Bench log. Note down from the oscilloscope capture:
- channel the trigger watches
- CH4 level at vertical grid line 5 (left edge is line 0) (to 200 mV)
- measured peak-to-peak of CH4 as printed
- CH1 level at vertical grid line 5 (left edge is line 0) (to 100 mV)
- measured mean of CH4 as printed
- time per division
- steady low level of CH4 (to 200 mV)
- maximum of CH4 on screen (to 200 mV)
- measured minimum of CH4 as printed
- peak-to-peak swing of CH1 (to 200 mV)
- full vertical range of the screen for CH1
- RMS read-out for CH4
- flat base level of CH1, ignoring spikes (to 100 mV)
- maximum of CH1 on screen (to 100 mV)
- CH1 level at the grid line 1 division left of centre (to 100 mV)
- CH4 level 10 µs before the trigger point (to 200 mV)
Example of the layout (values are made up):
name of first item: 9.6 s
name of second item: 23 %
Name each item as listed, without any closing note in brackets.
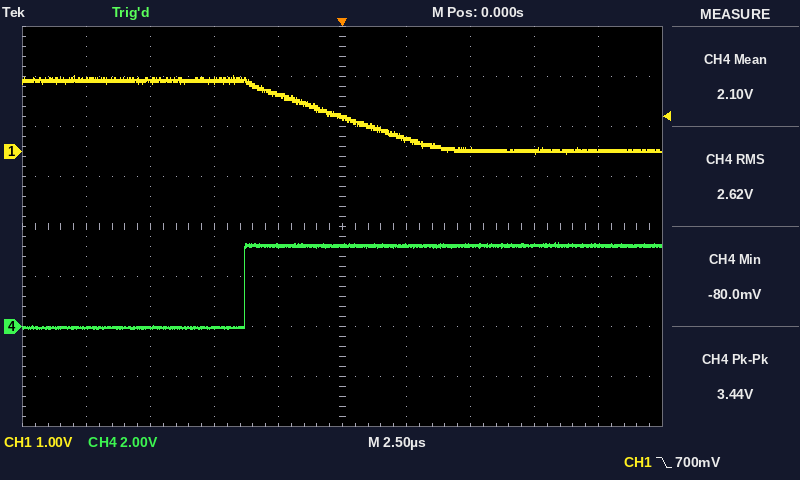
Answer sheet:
channel the trigger watches: CH1
CH4 level at vertical grid line 5 (left edge is line 0): 3.2 V
measured peak-to-peak of CH4 as printed: 3.44 V
CH1 level at vertical grid line 5 (left edge is line 0): 700 mV
measured mean of CH4 as printed: 2.10 V
time per division: 2.5 µs
steady low level of CH4: 0.0 V
maximum of CH4 on screen: 3.4 V
measured minimum of CH4 as printed: -80.0 mV
peak-to-peak swing of CH1: 1.6 V
full vertical range of the screen for CH1: 8 V
RMS read-out for CH4: 2.62 V
flat base level of CH1, ignoring spikes: 0.0 V
maximum of CH1 on screen: 1.5 V
CH1 level at the grid line 1 division left of centre: 1.2 V
CH4 level 10 µs before the trigger point: 0.0 V
